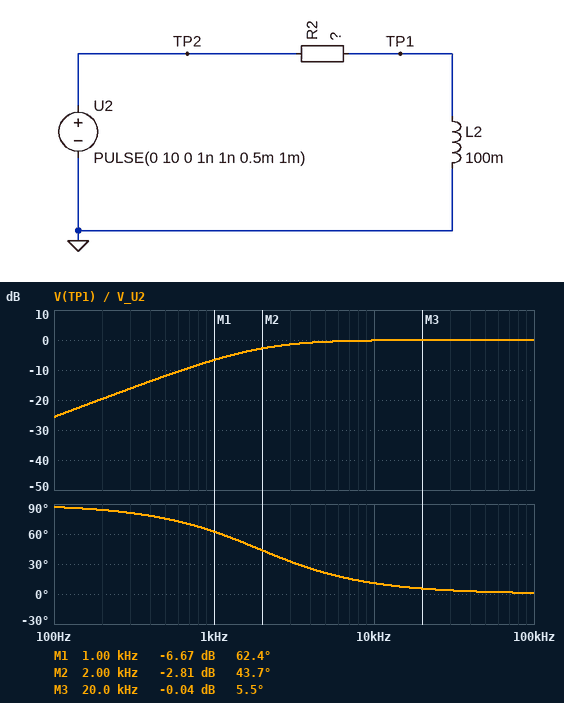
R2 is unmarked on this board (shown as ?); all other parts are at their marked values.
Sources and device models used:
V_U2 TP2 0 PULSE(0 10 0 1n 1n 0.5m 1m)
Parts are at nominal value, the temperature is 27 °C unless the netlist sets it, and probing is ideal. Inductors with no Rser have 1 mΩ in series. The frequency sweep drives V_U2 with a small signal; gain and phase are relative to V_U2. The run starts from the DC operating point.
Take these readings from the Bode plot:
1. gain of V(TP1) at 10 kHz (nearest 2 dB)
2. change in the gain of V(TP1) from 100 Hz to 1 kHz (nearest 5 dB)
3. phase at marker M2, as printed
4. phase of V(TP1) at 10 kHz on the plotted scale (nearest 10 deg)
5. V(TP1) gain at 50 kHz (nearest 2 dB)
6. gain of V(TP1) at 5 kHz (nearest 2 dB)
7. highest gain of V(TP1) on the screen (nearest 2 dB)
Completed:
0 dB
20 dB
43.7 deg
10 deg
0 dB
0 dB
0 dB
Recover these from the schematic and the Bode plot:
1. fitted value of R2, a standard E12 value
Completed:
1.2 kΩ
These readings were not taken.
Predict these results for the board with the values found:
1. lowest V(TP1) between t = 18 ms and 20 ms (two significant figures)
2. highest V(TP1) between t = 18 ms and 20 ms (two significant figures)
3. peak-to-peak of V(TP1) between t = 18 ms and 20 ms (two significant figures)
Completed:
-10 V
10 V
20 V
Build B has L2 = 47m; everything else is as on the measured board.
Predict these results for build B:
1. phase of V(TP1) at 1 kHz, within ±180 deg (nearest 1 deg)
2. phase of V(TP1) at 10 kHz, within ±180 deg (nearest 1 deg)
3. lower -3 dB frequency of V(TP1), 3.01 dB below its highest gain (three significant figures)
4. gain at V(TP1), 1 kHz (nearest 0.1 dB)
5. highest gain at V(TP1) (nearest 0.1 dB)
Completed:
76 deg
22 deg
4.06 kHz
-12.4 dB
0 dB
